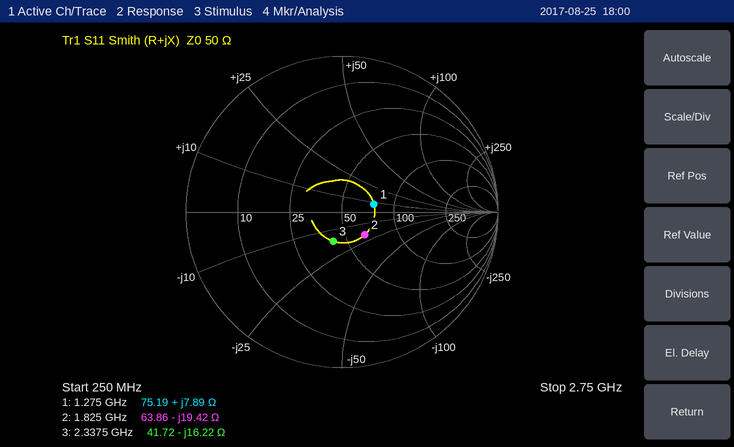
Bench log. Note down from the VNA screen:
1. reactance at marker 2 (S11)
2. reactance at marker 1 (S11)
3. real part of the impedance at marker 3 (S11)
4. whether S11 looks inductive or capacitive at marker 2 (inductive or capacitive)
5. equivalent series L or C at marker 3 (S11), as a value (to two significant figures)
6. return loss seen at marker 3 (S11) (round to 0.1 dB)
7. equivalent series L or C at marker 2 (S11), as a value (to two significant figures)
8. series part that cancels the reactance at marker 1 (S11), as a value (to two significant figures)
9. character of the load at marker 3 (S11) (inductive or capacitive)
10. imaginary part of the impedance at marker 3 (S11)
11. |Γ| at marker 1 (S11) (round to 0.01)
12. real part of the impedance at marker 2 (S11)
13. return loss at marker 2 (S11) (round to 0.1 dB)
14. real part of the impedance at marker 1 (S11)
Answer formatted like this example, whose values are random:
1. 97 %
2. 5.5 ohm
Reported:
1. -19.42 Ω
2. +7.89 Ω
3. 41.72 Ω
4. capacitive
5. 4.2 pF
6. 14.2 dB
7. 4.5 pF
8. 16 pF
9. capacitive
10. -16.22 Ω
11. 0.21
12. 63.86 Ω
13. 13.7 dB
14. 75.19 Ω
